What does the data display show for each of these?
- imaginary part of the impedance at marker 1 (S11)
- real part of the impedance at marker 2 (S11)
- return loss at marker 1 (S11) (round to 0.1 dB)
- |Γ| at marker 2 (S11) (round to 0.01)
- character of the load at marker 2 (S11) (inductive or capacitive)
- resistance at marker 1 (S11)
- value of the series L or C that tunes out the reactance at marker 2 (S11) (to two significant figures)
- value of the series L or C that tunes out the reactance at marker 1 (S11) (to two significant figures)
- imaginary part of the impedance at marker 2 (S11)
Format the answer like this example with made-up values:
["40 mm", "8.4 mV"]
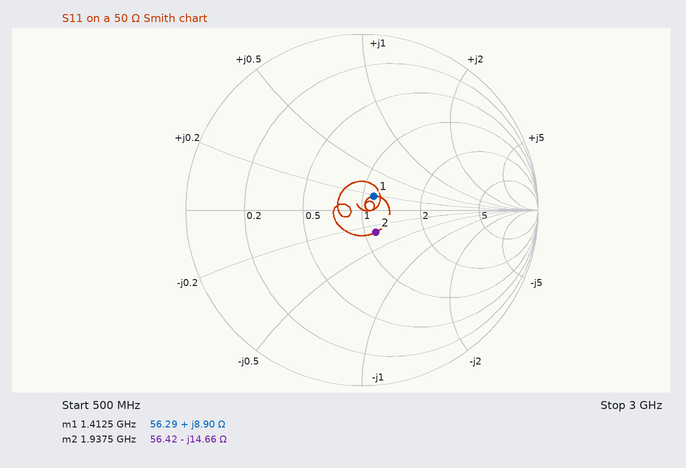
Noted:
["+8.90 Ω", "56.42 Ω", "19.8 dB", "0.15", "capacitive", "56.29 Ω", "1.2 nH", "13 pF", "-14.66 Ω"]
